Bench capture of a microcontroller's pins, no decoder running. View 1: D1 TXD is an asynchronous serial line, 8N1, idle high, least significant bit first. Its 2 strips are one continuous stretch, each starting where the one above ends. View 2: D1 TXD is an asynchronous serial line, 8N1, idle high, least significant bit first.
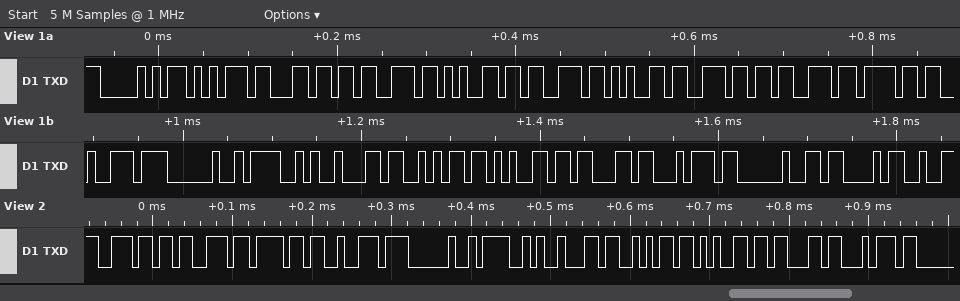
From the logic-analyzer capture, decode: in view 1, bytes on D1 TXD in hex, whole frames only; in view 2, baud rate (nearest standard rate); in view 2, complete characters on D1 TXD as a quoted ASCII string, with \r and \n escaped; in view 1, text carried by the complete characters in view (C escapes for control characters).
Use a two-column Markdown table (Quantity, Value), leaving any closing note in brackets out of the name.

| Quantity | Value |
|---|---|
| in view 1, bytes on D1 TXD in hex, whole frames only | 0x50 0x75 0x6C 0x73 0x65 0x73 0x65 0x6E 0x73 0x6F 0x72 0x20 0x4F 0x62 0x6A 0x65 0x63 0x74 0x20 0x43 |
| in view 2, baud rate | 115200 baud |
| in view 2, complete characters on D1 TXD as a quoted ASCII string, with \r and \n escaped | "nsor Object" |
| in view 1, text carried by the complete characters in view | "Pulsesensor Object C" |
